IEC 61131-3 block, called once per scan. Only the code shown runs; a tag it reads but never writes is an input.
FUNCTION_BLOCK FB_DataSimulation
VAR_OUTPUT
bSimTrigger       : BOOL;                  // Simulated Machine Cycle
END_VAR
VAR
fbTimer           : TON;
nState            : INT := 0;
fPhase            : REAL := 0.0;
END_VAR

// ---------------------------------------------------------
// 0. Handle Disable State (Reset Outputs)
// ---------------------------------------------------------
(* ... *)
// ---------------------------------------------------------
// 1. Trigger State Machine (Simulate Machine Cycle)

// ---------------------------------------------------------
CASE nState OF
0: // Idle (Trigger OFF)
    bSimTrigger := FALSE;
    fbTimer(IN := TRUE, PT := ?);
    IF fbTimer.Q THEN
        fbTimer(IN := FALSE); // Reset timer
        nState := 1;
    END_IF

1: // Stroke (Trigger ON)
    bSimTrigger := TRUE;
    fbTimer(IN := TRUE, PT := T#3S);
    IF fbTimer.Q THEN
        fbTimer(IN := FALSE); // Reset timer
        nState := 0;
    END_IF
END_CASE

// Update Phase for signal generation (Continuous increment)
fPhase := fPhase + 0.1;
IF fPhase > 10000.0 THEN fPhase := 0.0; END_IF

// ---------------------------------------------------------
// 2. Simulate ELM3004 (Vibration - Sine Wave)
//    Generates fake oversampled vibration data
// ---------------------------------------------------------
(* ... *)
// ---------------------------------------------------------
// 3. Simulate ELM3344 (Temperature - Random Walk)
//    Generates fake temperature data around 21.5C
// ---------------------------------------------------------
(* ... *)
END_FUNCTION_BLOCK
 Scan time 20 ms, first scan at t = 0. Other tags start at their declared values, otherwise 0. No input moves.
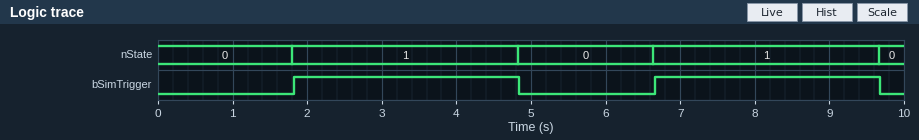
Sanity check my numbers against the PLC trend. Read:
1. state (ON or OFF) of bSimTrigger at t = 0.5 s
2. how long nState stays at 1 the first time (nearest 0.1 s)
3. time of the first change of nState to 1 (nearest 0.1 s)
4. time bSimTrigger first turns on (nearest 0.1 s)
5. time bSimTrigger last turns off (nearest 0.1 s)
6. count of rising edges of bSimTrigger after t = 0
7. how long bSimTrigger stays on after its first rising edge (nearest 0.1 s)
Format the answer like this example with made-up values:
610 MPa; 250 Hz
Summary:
OFF; 3.0 s; 1.8 s; 1.8 s; 9.7 s; 2; 3.0 s
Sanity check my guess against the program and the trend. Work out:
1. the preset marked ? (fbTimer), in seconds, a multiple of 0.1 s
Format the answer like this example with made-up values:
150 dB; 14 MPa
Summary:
1.8 s
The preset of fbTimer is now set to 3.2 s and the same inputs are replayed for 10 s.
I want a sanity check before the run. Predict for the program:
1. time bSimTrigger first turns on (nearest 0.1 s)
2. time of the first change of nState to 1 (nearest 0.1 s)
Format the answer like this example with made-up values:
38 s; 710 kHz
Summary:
3.2 s; 3.2 s
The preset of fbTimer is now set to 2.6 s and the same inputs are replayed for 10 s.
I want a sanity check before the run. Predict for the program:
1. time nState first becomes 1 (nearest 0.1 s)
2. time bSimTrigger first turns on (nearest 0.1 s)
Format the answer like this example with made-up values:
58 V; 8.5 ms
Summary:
2.6 s; 2.6 s
